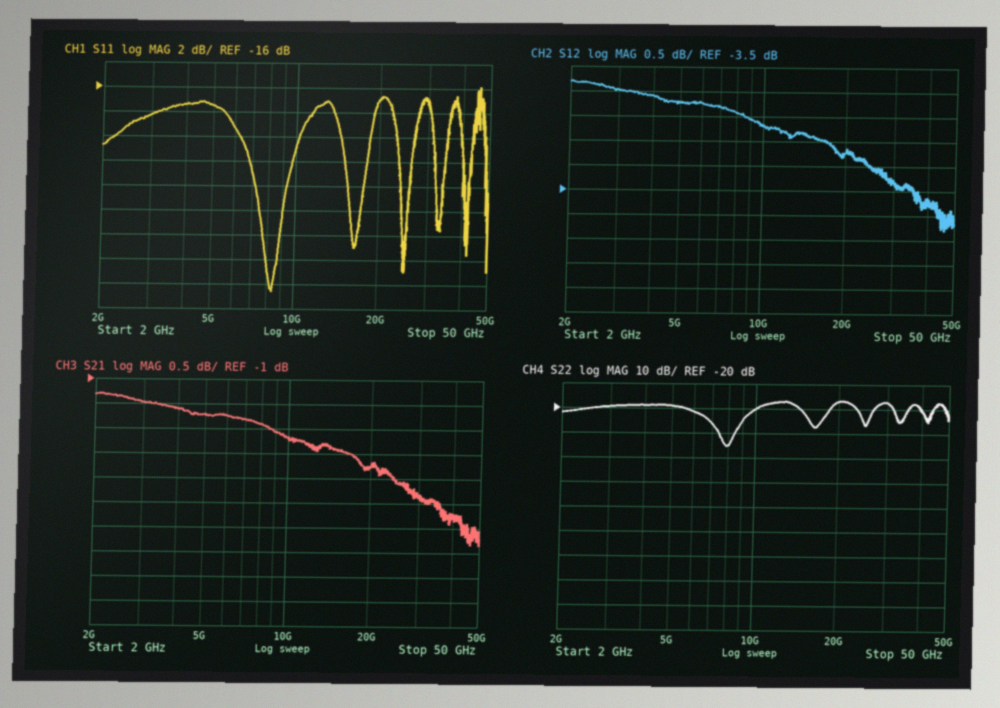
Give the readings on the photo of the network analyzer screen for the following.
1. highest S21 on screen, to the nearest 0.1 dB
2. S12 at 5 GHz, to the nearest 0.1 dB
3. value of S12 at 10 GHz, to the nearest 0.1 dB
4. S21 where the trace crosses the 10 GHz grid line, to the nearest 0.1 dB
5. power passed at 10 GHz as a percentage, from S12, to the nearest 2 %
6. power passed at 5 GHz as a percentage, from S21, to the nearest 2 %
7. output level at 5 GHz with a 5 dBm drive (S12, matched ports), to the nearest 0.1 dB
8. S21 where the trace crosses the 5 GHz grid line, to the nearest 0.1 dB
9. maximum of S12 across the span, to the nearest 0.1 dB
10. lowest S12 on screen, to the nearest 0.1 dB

-1.3 dB
-1.7 dB
-2.2 dB
-2.2 dB
60 %
68 %
3.3 dBm
-1.7 dB
-1.3 dB
-4.3 dB
